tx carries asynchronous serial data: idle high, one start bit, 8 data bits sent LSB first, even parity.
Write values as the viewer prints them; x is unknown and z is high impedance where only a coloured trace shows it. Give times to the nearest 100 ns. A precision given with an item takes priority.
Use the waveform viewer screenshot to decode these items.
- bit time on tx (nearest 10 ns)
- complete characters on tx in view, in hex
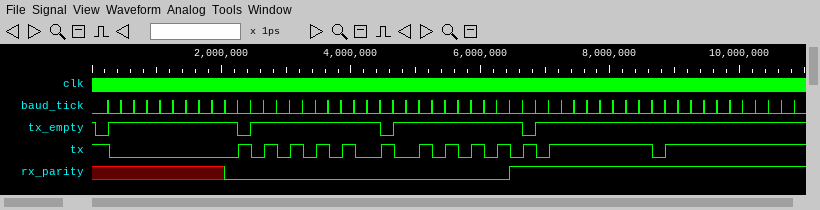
200 ns
00, 55, AA, FF
